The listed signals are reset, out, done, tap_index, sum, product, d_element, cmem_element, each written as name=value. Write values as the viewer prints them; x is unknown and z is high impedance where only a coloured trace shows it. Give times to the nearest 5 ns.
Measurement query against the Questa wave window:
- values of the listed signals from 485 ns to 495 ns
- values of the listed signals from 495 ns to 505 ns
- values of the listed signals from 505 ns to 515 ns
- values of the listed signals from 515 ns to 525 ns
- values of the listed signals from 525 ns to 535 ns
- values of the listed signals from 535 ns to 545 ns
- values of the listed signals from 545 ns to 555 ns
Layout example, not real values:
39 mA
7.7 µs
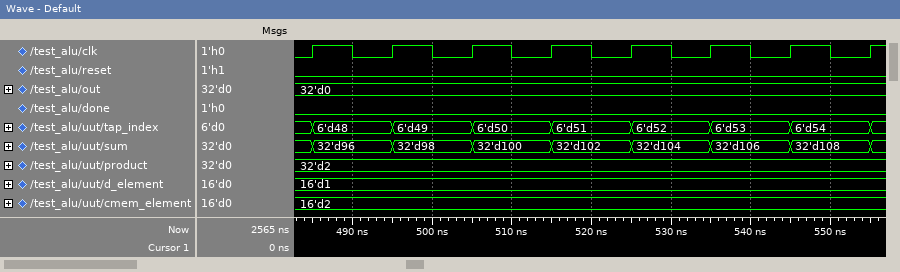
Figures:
reset=0, out=32'd0, done=0, tap_index=6'd48, sum=32'd96, product=32'd2, d_element=16'd1, cmem_element=16'd2
reset=0, out=32'd0, done=0, tap_index=6'd49, sum=32'd98, product=32'd2, d_element=16'd1, cmem_element=16'd2
reset=0, out=32'd0, done=0, tap_index=6'd50, sum=32'd100, product=32'd2, d_element=16'd1, cmem_element=16'd2
reset=0, out=32'd0, done=0, tap_index=6'd51, sum=32'd102, product=32'd2, d_element=16'd1, cmem_element=16'd2
reset=0, out=32'd0, done=0, tap_index=6'd52, sum=32'd104, product=32'd2, d_element=16'd1, cmem_element=16'd2
reset=0, out=32'd0, done=0, tap_index=6'd53, sum=32'd106, product=32'd2, d_element=16'd1, cmem_element=16'd2
reset=0, out=32'd0, done=0, tap_index=6'd54, sum=32'd108, product=32'd2, d_element=16'd1, cmem_element=16'd2
